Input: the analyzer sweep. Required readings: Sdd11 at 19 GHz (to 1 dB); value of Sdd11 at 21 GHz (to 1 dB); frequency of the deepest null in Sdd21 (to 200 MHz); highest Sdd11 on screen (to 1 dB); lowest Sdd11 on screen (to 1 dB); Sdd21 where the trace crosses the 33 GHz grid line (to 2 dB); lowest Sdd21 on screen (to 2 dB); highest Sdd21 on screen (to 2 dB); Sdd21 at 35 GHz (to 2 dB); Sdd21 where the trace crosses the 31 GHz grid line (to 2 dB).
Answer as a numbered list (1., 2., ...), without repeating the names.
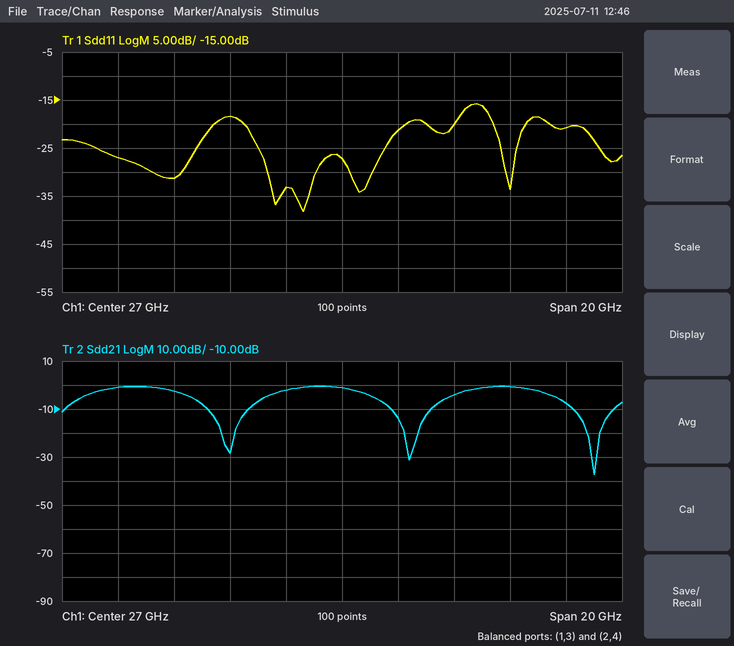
1. -27 dB
2. -31 dB
3. 36.0 GHz
4. -16 dB
5. -38 dB
6. 0 dB
7. -38 dB
8. 0 dB
9. -8 dB
10. -4 dB
